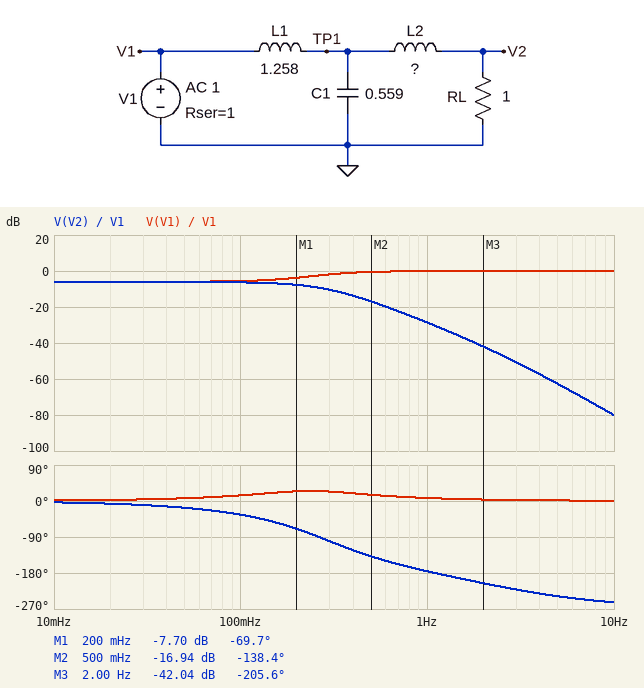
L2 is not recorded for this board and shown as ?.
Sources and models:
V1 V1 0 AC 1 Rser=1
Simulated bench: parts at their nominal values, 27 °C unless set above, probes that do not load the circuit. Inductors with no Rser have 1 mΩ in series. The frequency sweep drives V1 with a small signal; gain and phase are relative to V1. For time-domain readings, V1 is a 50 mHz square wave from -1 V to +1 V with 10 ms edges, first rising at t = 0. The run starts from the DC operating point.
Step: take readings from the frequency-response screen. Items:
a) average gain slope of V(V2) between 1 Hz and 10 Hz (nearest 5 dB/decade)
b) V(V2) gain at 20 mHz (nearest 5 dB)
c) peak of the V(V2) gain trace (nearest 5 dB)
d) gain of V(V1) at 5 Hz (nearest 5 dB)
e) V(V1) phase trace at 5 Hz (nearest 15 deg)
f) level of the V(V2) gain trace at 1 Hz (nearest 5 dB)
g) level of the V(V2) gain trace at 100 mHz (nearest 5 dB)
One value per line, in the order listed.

-50 dB/decade
-5 dB
-5 dB
0 dB
0 deg
-30 dB
-5 dB
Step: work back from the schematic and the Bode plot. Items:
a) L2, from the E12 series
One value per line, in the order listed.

56 mH
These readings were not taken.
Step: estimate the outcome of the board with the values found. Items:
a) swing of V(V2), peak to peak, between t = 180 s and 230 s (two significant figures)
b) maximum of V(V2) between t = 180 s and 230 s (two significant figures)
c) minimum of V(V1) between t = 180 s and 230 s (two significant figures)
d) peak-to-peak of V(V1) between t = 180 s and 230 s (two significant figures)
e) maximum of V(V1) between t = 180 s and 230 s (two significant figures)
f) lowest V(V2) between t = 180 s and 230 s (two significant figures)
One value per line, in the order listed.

1.0 V
520 mV
-1.5 V
3.0 V
1.5 V
-520 mV
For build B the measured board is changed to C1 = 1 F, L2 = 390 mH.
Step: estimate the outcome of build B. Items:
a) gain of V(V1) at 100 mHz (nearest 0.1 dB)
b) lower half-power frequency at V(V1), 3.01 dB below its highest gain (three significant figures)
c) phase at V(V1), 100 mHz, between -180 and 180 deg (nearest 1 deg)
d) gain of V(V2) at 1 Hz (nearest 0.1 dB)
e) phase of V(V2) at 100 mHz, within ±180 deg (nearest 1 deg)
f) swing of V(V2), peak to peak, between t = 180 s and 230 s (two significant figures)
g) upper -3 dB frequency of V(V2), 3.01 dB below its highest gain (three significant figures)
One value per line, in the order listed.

-5.9 dB
243 mHz
12 deg
-41.8 dB
-49 deg
1.1 V
235 mHz
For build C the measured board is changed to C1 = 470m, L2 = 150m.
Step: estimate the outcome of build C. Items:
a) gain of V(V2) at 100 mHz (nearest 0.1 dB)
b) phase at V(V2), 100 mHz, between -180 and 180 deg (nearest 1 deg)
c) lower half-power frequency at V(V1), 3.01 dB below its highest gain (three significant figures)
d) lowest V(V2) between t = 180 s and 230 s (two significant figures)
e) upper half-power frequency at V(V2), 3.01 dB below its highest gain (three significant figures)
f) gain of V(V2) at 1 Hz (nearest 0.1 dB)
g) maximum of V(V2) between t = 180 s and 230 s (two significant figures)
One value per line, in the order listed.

-6.4 dB
-34 deg
231 mHz
-500 mV
281 mHz
-28.4 dB
500 mV
